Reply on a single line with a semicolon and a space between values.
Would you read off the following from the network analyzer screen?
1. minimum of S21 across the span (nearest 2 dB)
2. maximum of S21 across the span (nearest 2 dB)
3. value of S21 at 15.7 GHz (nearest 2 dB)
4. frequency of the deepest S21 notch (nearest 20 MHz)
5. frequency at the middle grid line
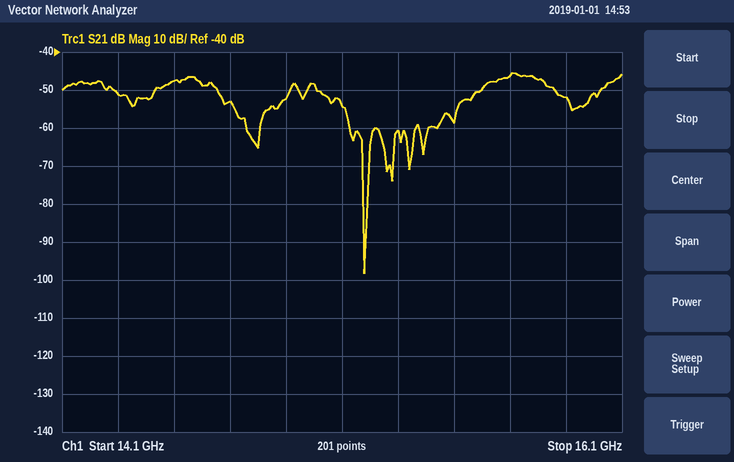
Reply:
-98 dB; -46 dB; -46 dB; 15.18 GHz; 15.1 GHz
